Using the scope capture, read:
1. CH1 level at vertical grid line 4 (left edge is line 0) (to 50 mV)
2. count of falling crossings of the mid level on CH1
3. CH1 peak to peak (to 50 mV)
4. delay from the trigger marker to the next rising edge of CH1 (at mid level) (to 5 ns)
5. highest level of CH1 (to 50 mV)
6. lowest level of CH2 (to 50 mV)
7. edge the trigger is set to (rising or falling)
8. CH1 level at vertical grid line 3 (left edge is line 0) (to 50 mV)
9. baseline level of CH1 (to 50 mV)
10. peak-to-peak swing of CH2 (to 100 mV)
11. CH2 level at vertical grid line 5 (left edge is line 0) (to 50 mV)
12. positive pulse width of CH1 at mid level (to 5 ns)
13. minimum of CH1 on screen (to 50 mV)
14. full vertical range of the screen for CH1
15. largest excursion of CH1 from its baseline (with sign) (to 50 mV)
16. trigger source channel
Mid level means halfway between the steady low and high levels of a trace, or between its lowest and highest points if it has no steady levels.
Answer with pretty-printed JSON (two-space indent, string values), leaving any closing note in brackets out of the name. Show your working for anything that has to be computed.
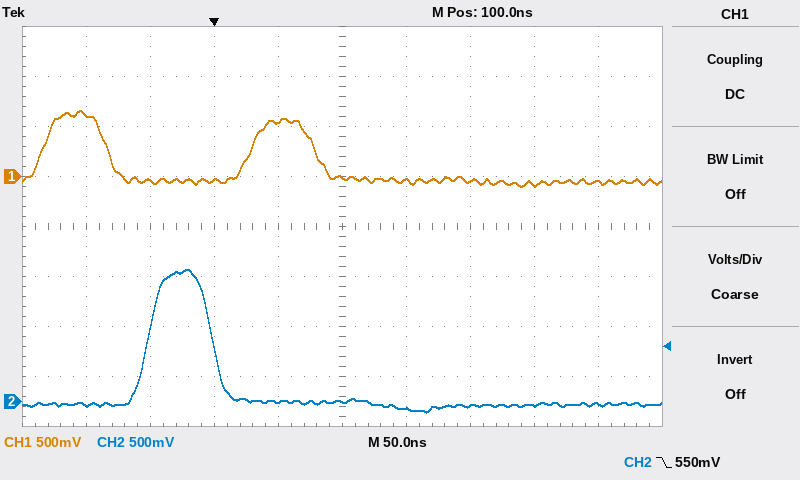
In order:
{
  "CH1 level at vertical grid line 4 (left edge is line 0)": "550 mV",
  "count of falling crossings of the mid level on CH1": "2",
  "CH1 peak to peak": "650 mV − (-100 mV) = 750 mV",
  "delay from the trigger marker to the next rising edge of CH1 (at mid level)": "30 ns",
  "highest level of CH1": "650 mV",
  "lowest level of CH2": "-100 mV",
  "edge the trigger is set to": "falling",
  "CH1 level at vertical grid line 3 (left edge is line 0)": "-50 mV",
  "baseline level of CH1": "-50 mV",
  "peak-to-peak swing of CH2": "1.40 V",
  "CH2 level at vertical grid line 5 (left edge is line 0)": "0 mV",
  "positive pulse width of CH1 at mid level": "50 ns",
  "minimum of CH1 on screen": "-100 mV",
  "full vertical range of the screen for CH1": "4 V",
  "largest excursion of CH1 from its baseline (with sign)": "650 mV − (-50 mV) = +700 mV",
  "trigger source channel": "CH2"
}
